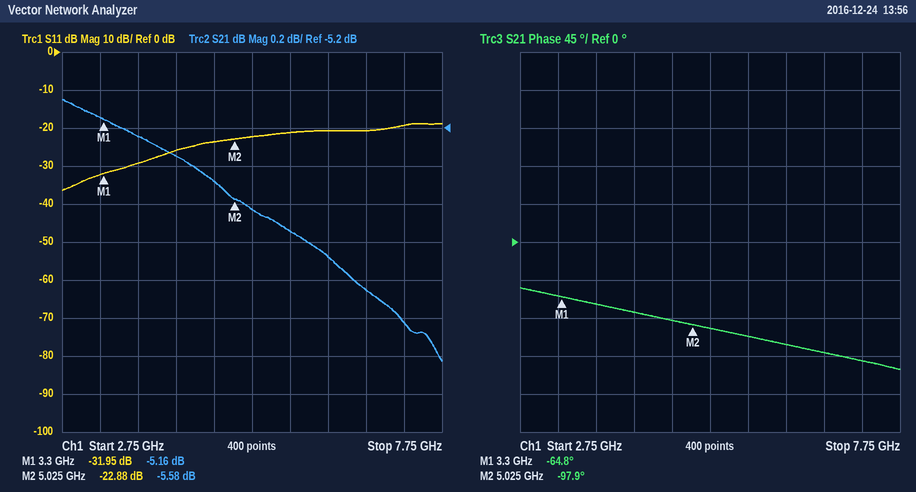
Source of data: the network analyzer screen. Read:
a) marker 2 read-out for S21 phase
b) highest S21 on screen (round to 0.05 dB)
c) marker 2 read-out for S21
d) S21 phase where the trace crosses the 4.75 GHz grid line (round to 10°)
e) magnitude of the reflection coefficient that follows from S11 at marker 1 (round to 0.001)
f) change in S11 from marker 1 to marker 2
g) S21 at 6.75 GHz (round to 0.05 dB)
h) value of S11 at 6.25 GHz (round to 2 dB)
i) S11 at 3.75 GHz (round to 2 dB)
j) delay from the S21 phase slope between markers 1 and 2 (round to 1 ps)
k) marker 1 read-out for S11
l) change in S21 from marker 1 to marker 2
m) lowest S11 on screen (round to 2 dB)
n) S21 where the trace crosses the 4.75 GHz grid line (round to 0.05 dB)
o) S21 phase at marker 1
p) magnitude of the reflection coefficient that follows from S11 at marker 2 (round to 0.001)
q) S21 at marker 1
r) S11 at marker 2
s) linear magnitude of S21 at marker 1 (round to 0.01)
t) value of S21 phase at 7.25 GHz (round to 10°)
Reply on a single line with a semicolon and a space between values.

-97.9°; -5.05 dB; -5.58 dB; -90°; 0.025; 9.07 dB; -6.05 dB; -20 dB; -30 dB; 53 ps; -31.95 dB; -0.42 dB; -36 dB; -5.50 dB; -64.8°; 0.072; -5.16 dB; -22.88 dB; 0.55; -140°
